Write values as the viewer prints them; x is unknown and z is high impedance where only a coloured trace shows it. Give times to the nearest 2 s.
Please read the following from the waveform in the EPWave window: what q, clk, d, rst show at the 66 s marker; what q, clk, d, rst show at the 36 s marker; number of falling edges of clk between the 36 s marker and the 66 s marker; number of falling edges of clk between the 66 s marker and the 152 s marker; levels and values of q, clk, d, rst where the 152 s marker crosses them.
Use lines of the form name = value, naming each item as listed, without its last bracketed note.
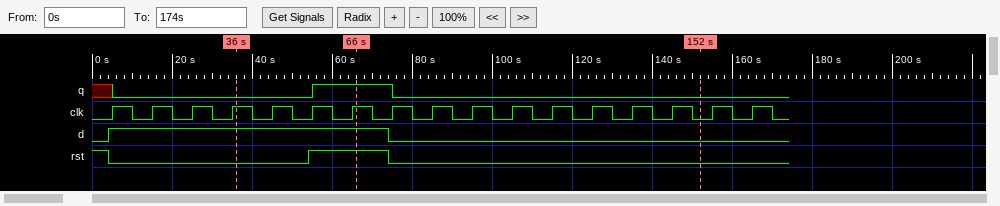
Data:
what q, clk, d, rst show at the 66 s marker = q=1, clk=1, d=1, rst=1
what q, clk, d, rst show at the 36 s marker = q=0, clk=1, d=1, rst=0
number of falling edges of clk between the 36 s marker and the 66 s marker = 3
number of falling edges of clk between the 66 s marker and the 152 s marker = 9
levels and values of q, clk, d, rst where the 152 s marker crosses them = q=0, clk=0, d=0, rst=0
